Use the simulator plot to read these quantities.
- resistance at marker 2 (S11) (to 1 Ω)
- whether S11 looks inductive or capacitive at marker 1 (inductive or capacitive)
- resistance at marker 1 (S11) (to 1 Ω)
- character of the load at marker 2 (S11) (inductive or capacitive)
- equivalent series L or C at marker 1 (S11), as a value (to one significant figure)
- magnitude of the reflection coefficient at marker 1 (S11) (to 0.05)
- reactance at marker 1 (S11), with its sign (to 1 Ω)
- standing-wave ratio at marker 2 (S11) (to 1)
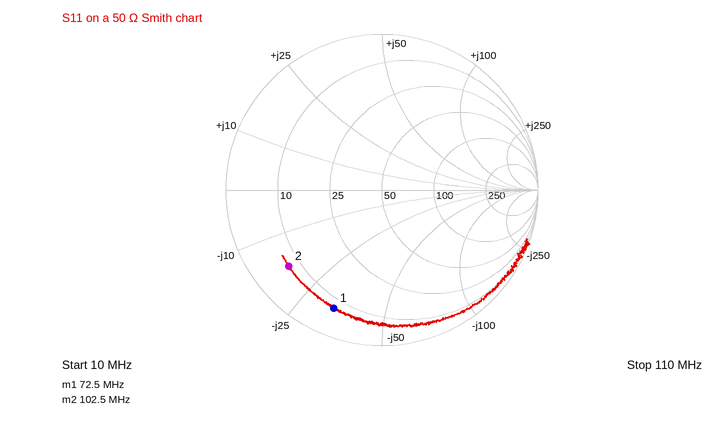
7 Ω
capacitive
7 Ω
capacitive
70 pF
0.80
-33 Ω
8
